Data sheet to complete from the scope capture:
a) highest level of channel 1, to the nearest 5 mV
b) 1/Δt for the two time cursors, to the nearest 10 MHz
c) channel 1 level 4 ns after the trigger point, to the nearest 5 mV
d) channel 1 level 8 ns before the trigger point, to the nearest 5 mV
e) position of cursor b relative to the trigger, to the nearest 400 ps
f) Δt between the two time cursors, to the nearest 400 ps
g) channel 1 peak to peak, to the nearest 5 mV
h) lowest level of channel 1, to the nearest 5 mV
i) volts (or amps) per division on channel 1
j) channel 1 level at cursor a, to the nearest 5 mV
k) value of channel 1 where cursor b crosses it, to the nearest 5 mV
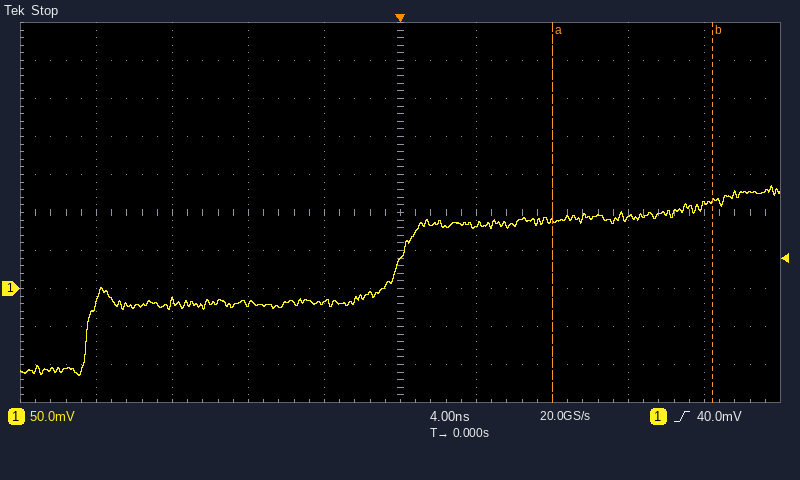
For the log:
135 mV
120 MHz
85 mV
-20 mV
+16.4 ns
8.4 ns
250 mV
-115 mV
50 mV
90 mV
115 mV
